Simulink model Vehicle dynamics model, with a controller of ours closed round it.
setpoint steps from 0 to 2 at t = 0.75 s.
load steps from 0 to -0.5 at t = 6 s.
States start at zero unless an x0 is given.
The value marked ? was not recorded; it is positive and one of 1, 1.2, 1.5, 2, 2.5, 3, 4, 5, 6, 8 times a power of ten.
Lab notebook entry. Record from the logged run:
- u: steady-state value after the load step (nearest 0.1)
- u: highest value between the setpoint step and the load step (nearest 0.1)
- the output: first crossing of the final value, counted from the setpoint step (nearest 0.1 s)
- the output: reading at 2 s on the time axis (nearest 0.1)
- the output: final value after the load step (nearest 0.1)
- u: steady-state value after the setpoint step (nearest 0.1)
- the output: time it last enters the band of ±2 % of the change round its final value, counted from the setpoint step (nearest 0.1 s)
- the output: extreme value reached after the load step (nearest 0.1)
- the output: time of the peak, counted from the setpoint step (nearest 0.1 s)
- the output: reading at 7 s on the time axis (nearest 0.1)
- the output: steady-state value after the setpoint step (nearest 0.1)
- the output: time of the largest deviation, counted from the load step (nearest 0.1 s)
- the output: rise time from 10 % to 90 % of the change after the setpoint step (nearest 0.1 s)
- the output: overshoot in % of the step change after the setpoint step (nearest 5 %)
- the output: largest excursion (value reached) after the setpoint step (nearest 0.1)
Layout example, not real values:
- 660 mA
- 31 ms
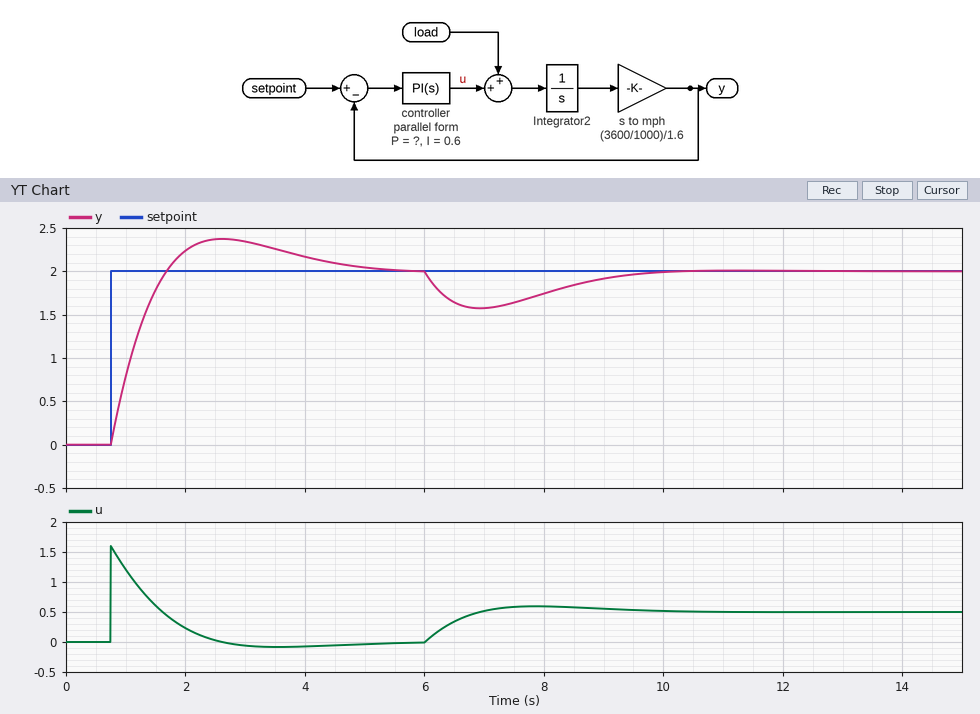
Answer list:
- 0.5
- 1.6
- 0.9 s
- 2.2
- 2.0
- 0.0
- 4.3 s
- 1.6
- 1.9 s
- 1.6
- 2.0
- 0.9 s
- 0.7 s
- 20 %
- 2.4
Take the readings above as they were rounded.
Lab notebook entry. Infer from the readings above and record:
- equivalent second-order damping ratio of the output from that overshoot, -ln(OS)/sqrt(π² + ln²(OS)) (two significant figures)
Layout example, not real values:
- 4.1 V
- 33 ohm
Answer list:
- 0.46
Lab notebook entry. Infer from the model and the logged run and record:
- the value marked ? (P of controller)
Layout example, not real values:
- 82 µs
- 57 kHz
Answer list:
- 0.8
